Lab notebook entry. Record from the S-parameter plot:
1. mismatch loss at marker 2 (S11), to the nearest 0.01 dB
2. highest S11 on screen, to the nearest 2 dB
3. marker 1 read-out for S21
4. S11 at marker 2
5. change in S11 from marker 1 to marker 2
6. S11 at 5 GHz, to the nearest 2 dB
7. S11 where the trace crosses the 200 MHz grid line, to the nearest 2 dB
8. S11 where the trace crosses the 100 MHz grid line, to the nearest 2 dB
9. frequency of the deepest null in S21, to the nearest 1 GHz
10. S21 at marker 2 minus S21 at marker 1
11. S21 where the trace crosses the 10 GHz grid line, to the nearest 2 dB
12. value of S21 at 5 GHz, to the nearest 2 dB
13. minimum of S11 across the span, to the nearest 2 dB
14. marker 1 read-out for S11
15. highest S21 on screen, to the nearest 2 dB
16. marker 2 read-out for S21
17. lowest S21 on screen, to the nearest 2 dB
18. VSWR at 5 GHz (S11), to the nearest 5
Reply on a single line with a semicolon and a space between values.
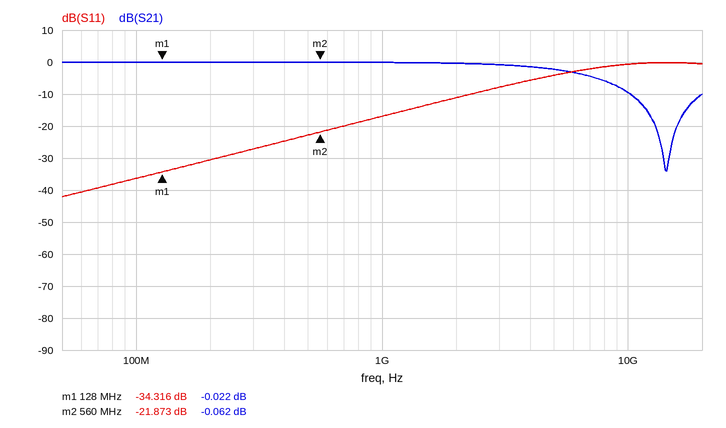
0.03 dB; 0 dB; -0.022 dB; -21.873 dB; 12.443 dB; -4 dB; -30 dB; -36 dB; 14 GHz; -0.040 dB; -10 dB; -2 dB; -42 dB; -34.316 dB; 0 dB; -0.062 dB; -34 dB; 5
